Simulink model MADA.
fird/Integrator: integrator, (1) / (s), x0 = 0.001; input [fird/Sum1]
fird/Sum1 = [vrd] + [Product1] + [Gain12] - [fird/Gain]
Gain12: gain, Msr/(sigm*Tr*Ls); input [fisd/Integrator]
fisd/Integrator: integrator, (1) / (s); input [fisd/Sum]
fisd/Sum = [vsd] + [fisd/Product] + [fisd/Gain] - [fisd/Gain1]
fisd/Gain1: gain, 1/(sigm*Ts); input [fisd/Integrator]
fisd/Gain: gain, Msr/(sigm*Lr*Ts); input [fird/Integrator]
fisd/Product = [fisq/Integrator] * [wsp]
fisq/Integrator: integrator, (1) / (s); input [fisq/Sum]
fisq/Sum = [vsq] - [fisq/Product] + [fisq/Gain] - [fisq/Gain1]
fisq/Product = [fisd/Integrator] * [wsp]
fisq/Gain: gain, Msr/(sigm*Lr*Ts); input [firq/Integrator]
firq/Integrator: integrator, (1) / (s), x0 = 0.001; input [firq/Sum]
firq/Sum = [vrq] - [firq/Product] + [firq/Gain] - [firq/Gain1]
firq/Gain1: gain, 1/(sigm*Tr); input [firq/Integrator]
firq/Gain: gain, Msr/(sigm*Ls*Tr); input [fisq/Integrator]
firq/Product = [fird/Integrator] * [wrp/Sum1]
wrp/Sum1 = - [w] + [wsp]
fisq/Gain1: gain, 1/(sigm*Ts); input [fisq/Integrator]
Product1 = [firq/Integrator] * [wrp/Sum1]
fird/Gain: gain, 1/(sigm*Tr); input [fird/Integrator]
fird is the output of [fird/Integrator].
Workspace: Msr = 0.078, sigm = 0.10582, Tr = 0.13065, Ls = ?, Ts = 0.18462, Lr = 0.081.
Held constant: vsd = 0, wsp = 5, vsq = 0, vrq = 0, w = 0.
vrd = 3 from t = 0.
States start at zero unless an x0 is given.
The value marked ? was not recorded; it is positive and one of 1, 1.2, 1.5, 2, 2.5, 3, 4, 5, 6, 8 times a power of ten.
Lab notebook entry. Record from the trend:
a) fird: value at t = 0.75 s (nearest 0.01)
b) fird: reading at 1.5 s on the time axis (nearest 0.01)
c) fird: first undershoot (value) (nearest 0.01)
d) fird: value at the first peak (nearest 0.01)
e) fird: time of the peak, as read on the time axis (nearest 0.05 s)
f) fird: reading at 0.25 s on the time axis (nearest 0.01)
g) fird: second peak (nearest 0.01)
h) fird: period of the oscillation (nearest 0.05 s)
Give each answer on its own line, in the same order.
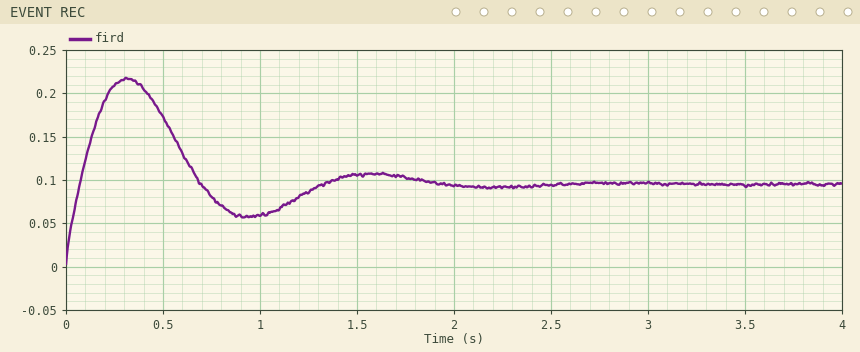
0.08
0.11
0.06
0.22
0.30 s
0.21
0.11
1.25 s
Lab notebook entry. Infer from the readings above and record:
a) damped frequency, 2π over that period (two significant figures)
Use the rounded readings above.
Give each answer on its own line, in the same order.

5.0 rad/s
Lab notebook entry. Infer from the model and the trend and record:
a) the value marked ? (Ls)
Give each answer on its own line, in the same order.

0.08
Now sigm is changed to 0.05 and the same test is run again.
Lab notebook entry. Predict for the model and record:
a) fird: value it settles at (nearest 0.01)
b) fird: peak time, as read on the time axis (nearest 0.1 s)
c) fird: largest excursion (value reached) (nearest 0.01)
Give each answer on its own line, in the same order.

0.13
0.3 s
0.17
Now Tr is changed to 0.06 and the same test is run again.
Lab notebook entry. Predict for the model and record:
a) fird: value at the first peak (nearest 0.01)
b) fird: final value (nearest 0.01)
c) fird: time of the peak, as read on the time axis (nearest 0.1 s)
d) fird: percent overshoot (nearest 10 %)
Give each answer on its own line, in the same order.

0.12
0.07
0.3 s
80 %
